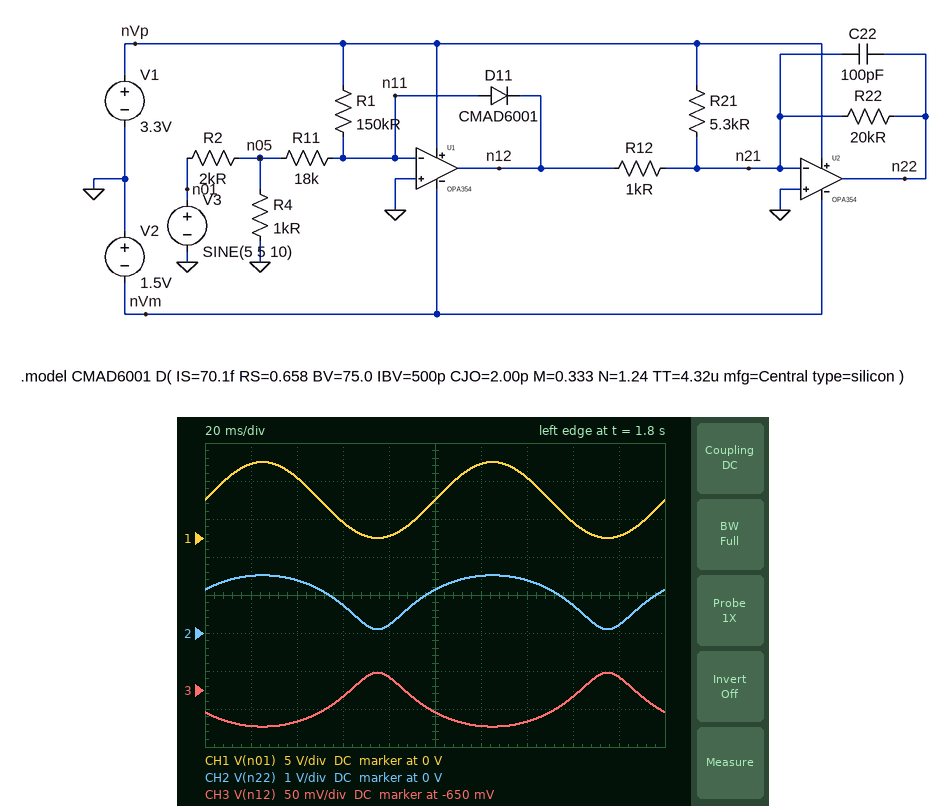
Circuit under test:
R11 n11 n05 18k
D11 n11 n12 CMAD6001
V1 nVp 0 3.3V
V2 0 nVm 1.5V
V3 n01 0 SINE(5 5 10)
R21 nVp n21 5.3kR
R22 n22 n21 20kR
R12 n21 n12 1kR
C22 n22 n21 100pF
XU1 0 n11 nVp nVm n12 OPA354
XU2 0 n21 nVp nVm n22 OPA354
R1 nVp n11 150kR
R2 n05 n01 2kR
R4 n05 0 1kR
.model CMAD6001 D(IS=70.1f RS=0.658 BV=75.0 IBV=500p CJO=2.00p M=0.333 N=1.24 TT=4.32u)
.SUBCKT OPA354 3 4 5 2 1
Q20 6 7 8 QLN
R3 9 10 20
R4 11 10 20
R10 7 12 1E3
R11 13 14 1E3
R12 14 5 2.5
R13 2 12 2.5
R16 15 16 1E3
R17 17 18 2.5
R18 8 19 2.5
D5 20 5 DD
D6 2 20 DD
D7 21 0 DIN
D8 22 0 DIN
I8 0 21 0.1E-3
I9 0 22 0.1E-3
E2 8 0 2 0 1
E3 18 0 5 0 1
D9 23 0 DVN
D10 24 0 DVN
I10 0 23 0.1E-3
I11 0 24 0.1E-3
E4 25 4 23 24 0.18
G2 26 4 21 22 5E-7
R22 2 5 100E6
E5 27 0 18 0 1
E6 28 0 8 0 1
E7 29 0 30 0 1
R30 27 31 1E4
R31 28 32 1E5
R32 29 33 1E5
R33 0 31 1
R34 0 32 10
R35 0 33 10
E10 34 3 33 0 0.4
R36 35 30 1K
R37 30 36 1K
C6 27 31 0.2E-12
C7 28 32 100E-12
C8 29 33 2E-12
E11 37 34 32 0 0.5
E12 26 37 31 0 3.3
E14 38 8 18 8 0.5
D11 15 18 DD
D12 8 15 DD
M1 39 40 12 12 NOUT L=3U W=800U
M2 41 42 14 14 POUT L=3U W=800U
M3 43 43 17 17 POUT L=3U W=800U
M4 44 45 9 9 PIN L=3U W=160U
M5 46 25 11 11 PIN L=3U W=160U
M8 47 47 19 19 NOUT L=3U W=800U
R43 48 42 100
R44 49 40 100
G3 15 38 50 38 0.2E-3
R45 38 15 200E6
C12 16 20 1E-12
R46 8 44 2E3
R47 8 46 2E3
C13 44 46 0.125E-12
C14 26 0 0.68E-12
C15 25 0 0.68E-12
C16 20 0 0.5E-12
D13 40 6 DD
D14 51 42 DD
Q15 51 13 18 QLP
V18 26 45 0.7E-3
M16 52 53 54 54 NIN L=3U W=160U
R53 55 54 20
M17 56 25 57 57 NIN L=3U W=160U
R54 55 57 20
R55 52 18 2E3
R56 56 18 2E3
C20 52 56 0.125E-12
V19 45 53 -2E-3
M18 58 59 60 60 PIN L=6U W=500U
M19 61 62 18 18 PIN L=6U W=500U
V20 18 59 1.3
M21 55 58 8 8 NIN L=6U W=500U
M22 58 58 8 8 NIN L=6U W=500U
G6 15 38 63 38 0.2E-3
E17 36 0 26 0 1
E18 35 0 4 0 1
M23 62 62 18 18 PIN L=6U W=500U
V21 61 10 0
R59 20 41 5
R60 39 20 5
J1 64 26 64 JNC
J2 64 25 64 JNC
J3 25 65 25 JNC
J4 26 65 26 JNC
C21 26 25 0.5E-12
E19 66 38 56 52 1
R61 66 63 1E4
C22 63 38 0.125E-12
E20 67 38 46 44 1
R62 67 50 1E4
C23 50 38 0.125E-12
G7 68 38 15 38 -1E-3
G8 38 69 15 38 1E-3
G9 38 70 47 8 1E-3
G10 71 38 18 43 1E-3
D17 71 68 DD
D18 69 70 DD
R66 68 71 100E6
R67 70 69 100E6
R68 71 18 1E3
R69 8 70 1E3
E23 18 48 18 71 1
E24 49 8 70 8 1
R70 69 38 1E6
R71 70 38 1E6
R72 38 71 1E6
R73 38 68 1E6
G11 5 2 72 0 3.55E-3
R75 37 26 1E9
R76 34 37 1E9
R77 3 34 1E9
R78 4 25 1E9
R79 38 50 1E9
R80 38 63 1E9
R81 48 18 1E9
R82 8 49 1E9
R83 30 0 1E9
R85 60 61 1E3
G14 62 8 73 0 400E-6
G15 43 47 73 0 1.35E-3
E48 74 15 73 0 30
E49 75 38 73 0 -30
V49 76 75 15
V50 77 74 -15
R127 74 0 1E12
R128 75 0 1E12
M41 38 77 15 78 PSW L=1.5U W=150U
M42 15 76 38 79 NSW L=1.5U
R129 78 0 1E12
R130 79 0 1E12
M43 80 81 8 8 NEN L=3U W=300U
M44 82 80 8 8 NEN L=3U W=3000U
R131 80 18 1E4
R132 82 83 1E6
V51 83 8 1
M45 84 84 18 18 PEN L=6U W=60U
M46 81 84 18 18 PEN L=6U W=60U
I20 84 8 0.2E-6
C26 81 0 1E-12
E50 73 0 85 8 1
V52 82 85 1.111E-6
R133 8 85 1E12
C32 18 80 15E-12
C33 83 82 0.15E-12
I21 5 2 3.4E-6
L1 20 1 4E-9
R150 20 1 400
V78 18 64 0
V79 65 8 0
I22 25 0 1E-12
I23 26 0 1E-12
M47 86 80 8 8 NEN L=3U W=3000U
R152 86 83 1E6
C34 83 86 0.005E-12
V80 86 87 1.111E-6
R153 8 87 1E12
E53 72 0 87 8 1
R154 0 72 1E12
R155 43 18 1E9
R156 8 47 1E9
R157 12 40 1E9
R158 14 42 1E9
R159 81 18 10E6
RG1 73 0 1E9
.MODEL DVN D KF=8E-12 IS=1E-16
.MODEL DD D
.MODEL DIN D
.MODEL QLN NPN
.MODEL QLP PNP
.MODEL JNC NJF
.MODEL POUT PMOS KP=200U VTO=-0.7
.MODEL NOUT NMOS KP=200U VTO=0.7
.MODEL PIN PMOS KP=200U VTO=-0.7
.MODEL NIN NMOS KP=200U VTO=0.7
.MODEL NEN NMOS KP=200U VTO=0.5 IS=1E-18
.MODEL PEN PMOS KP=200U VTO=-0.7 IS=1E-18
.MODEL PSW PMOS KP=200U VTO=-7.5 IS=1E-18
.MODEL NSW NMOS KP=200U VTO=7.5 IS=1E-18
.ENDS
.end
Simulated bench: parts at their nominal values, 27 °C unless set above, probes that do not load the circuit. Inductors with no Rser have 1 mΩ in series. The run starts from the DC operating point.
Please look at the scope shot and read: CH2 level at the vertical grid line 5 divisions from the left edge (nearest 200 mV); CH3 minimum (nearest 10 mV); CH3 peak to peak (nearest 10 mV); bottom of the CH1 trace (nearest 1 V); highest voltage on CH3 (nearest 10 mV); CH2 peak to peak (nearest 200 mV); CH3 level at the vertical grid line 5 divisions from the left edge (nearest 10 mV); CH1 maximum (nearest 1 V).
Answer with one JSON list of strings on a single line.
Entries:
["1.2 V", "-700 mV", "70 mV", "0 V", "-630 mV", "1.4 V", "-680 mV", "10 V"]
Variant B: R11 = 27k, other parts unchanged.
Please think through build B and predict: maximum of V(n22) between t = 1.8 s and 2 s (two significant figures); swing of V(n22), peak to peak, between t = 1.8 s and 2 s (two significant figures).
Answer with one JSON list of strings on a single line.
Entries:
["1.3 V", "1.2 V"]
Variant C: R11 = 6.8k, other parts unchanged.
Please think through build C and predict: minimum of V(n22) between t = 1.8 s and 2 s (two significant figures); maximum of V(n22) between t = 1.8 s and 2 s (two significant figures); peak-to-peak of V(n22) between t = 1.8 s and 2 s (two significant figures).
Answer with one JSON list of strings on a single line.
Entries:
["97 mV", "2.1 V", "2.0 V"]
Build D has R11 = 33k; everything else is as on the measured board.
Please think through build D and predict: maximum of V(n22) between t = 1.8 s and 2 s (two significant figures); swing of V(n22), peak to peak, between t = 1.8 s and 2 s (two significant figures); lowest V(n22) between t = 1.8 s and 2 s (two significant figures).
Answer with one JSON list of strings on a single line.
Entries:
["1.2 V", "1.1 V", "98 mV"]
